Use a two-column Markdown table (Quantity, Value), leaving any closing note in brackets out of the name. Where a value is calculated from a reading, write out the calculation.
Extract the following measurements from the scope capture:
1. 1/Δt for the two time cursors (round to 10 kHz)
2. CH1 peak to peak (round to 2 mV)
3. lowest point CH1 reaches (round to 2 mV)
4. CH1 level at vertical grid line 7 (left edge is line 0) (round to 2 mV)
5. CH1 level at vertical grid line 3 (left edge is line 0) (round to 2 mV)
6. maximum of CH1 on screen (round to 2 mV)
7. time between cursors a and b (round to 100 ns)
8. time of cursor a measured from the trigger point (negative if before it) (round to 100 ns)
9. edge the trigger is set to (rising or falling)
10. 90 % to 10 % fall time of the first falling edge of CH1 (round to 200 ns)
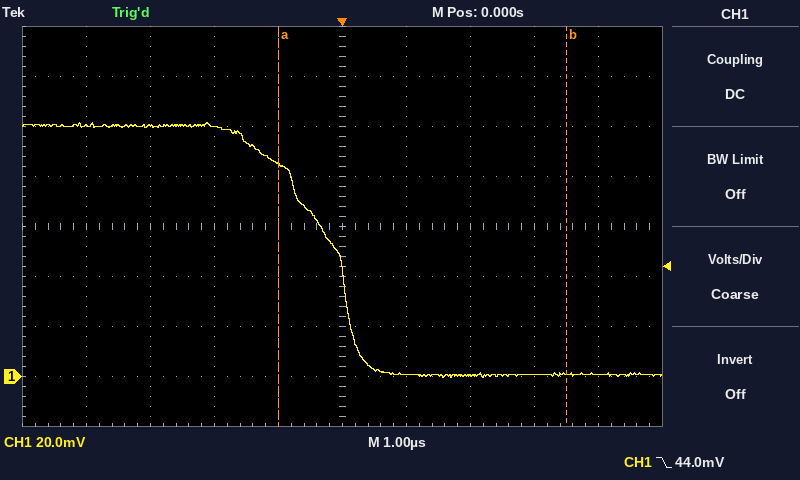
| Quantity | Value |
|---|---|
| 1/Δt for the two time cursors | 1 / 4.5 µs ≈ 220 kHz |
| CH1 peak to peak | 102 mV − (0 mV) = 102 mV |
| lowest point CH1 reaches | 0 mV |
| CH1 level at vertical grid line 7 (left edge is line 0) | 0 mV |
| CH1 level at vertical grid line 3 (left edge is line 0) | 100 mV |
| maximum of CH1 on screen | 102 mV |
| time between cursors a and b | 4.5 µs |
| time of cursor a measured from the trigger point (negative if before it) | -1.0 µs |
| edge the trigger is set to | falling |
| 90 % to 10 % fall time of the first falling edge of CH1 | 1.6 µs |
